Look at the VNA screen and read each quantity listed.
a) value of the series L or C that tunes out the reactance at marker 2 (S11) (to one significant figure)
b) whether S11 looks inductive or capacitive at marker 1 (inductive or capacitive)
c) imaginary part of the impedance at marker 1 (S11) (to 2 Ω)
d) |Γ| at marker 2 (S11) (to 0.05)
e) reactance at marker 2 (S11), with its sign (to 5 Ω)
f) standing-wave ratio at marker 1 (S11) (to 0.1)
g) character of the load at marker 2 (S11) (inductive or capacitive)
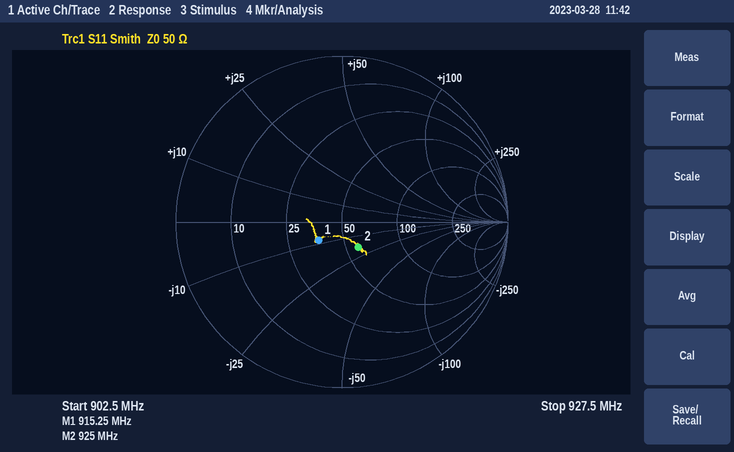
3 nH
capacitive
-8 Ω
0.20
-20 Ω
1.4
capacitive
